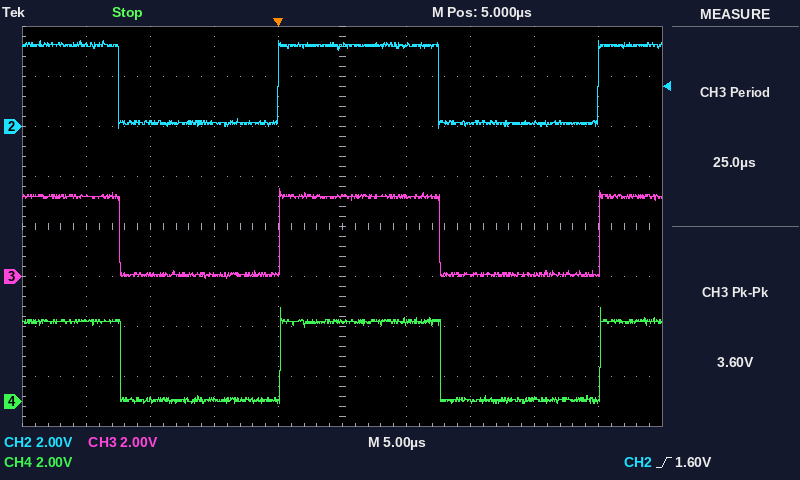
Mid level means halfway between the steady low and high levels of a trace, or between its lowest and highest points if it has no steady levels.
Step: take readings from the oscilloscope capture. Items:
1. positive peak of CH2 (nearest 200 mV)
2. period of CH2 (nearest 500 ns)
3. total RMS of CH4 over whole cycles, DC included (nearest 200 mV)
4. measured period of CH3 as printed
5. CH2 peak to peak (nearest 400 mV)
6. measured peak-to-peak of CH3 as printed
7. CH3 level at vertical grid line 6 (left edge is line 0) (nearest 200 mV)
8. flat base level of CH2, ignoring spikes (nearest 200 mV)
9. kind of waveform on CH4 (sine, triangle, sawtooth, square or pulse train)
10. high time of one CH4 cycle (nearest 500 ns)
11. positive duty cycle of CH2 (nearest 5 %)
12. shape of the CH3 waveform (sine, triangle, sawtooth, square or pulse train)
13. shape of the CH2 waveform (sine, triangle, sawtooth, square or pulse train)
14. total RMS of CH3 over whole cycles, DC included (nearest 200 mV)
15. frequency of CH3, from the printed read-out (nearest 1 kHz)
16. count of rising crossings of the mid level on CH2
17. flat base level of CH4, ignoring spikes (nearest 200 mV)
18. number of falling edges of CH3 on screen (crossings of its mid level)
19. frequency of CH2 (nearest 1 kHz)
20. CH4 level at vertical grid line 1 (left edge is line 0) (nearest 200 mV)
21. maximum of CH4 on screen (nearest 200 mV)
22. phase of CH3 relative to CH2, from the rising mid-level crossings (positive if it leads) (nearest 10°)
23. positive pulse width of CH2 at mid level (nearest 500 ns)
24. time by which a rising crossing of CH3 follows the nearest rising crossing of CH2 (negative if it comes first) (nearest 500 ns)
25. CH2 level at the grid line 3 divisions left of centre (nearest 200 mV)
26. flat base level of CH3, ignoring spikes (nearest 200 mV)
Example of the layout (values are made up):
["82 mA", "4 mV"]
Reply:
["3.4 V", "25.0 µs", "2.2 V", "25.0 µs", "3.6 V", "3.60 V", "3.2 V", "200 mV", "square", "12.5 µs", "50 %", "square", "square", "2.2 V", "40 kHz", "2", "0.0 V", "2", "40 kHz", "3.2 V", "3.8 V", "0°", "12.5 µs", "0.0 µs", "200 mV", "0.0 V"]
